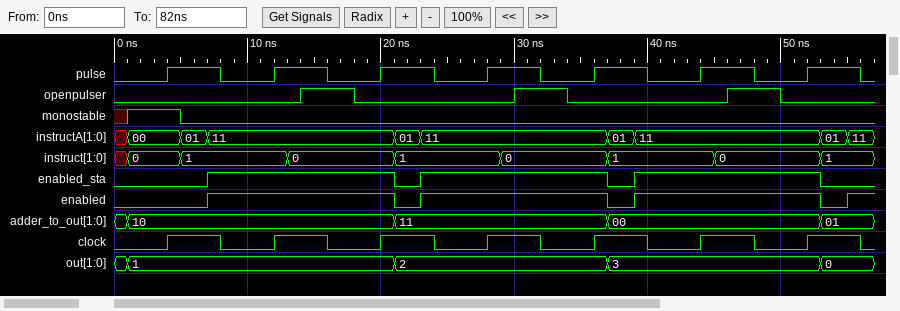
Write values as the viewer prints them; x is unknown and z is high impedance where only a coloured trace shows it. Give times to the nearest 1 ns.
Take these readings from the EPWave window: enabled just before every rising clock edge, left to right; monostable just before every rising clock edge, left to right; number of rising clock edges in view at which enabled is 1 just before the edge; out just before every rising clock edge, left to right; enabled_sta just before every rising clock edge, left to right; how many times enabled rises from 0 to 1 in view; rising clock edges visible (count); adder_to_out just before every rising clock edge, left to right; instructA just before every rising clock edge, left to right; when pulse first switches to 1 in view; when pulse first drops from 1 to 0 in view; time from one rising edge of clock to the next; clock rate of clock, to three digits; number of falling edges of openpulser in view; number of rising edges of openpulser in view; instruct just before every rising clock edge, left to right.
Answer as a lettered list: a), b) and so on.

a) 0 1 1 1 1 1 1
b) 1 0 0 0 0 0 0
c) 6
d) 1, 1, 1, 2, 2, 3, 3
e) 0 1 1 1 1 1 1
f) 4
g) 7
h) 10, 10, 10, 11, 11, 00, 00
i) 00, 11, 11, 11, 11, 11, 11
j) 4 ns
k) 8 ns
l) 8 ns
m) 125 MHz
n) 3
o) 3
p) 0, 1, 0, 1, 0, 1, 0
